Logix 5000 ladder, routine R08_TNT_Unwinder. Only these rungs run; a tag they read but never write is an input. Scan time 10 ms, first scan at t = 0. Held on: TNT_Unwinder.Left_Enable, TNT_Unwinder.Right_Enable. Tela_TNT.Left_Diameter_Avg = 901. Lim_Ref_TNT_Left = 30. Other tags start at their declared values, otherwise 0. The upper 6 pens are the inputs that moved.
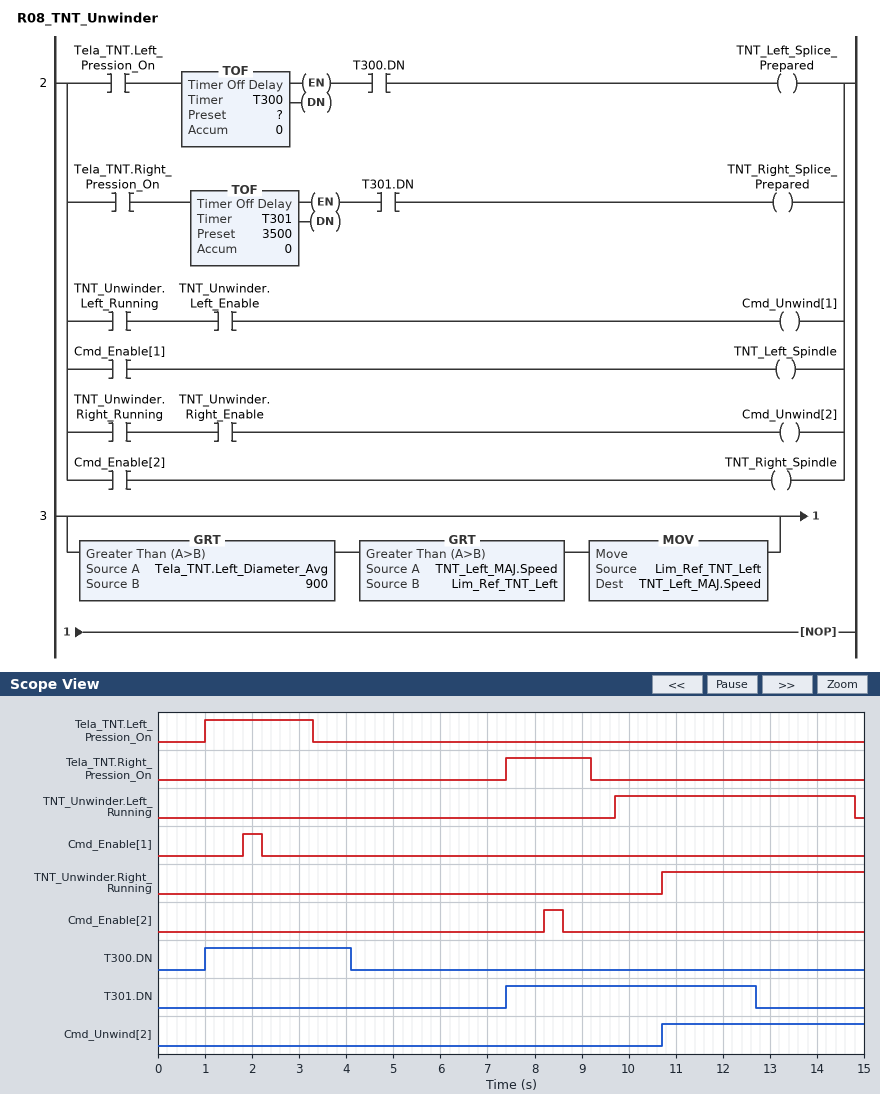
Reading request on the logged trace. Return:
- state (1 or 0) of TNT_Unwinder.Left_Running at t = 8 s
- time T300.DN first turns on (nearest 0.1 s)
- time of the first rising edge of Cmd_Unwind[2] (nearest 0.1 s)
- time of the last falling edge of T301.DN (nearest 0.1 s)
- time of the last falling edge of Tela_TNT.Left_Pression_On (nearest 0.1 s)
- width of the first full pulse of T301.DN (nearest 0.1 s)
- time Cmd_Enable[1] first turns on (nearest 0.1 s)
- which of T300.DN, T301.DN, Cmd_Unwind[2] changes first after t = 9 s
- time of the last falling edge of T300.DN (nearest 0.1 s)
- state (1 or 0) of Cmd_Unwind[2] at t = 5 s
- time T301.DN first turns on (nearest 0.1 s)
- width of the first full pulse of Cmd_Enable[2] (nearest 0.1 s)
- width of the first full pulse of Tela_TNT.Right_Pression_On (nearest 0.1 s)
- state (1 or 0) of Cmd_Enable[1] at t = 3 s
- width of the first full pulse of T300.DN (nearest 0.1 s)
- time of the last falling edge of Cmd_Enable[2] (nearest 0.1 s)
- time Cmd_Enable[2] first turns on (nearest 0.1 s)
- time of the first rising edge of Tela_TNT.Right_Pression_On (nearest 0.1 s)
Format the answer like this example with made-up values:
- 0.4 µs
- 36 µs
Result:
- 0
- 1.0 s
- 10.7 s
- 12.7 s
- 3.3 s
- 5.3 s
- 1.8 s
- Cmd_Unwind[2]
- 4.1 s
- 0
- 7.4 s
- 0.4 s
- 1.8 s
- 0
- 3.1 s
- 8.6 s
- 8.2 s
- 7.4 s
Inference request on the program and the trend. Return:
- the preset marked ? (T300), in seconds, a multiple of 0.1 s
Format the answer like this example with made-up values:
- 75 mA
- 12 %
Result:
- 0.8 s
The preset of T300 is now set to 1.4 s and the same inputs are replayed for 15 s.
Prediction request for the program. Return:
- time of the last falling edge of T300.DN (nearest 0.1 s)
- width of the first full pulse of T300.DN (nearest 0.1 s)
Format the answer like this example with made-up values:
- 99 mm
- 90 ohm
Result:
- 4.7 s
- 3.7 s
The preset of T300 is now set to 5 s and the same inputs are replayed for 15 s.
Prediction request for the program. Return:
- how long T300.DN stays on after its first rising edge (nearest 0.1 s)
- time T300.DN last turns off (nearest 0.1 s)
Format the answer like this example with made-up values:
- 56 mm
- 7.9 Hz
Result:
- 7.3 s
- 8.3 s
